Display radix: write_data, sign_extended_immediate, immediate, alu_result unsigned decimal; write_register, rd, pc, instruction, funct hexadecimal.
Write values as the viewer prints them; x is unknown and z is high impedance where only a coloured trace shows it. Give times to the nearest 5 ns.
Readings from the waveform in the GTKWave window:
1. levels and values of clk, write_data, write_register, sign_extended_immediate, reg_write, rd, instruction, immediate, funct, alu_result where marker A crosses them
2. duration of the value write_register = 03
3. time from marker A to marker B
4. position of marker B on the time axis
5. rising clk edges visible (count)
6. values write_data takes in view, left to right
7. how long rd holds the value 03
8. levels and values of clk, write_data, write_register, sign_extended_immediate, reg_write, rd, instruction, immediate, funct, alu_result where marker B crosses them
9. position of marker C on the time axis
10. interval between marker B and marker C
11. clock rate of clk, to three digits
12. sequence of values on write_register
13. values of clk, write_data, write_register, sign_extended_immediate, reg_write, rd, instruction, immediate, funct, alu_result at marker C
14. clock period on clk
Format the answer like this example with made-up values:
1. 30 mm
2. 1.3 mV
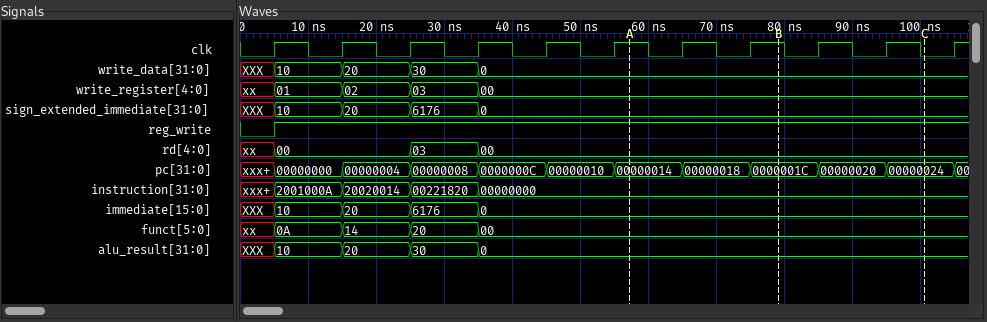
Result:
1. clk=1, write_data=0, write_register=00, sign_extended_immediate=0, reg_write=1, rd=00, instruction=00000000, immediate=0, funct=00, alu_result=0
2. 10 ns
3. 20 ns
4. 80 ns
5. 11
6. XXX, 10, 20, 30, 0
7. 10 ns
8. clk=1, write_data=0, write_register=00, sign_extended_immediate=0, reg_write=1, rd=00, instruction=00000000, immediate=0, funct=00, alu_result=0
9. 100 ns
10. 20 ns
11. 100 MHz
12. xx, 01, 02, 03, 00
13. clk=0, write_data=0, write_register=00, sign_extended_immediate=0, reg_write=1, rd=00, instruction=00000000, immediate=0, funct=00, alu_result=0
14. 10 ns
